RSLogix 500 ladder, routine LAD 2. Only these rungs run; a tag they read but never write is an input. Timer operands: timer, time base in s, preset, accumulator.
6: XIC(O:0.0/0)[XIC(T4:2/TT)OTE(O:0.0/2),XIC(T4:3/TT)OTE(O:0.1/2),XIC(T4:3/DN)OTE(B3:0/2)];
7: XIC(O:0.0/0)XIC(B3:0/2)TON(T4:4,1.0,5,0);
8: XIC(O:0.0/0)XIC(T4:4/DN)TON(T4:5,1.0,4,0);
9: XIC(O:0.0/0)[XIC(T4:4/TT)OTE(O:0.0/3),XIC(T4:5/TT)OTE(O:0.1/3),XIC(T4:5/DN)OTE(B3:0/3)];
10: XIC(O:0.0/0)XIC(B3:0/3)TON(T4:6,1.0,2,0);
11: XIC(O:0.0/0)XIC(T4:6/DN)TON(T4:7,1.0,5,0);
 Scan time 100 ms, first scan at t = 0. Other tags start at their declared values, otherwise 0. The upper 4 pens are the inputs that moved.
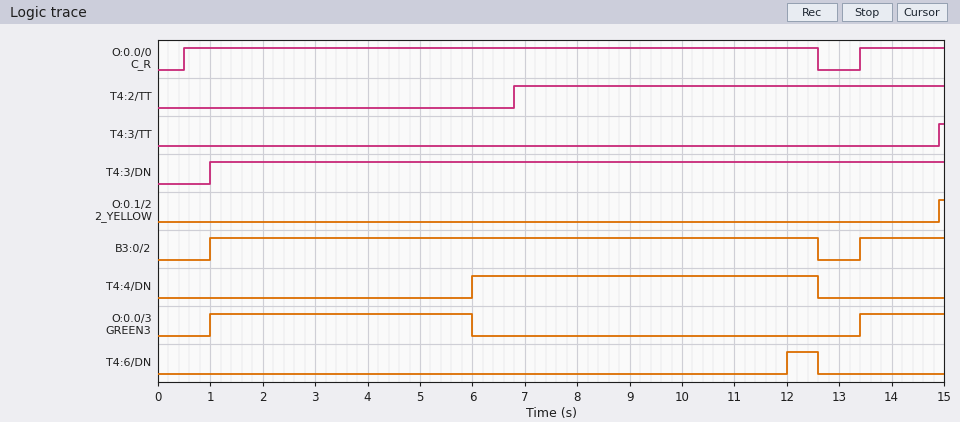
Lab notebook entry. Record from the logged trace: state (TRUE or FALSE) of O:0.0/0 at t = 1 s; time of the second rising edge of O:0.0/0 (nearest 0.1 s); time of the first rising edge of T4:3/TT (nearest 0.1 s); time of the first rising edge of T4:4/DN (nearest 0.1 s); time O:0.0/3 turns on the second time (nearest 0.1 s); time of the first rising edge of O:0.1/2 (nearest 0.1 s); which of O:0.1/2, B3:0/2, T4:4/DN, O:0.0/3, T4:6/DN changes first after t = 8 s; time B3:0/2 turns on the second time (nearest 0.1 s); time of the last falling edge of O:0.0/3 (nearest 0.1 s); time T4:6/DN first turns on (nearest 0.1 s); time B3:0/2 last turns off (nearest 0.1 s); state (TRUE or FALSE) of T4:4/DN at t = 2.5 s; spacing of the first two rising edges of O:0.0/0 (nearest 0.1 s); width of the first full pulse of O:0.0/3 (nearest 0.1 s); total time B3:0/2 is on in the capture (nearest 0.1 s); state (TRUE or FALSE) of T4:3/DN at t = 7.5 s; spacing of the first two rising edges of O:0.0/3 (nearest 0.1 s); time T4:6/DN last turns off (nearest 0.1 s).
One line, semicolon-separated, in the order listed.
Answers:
TRUE; 13.4 s; 14.9 s; 6.0 s; 13.4 s; 14.9 s; T4:6/DN; 13.4 s; 6.0 s; 12.0 s; 12.6 s; FALSE; 12.9 s; 5.0 s; 13.2 s; TRUE; 12.4 s; 12.6 s
